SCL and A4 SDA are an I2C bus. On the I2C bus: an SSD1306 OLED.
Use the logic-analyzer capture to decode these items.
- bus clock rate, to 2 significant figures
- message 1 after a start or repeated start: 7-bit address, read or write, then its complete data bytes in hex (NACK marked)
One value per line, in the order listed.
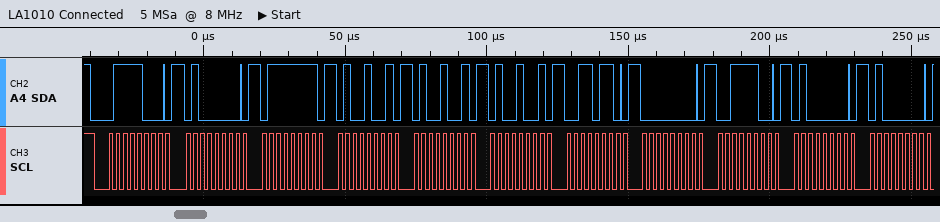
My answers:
400 kHz
0x3C write: 40 7F 49 49 49 36 00 3C 40 40
